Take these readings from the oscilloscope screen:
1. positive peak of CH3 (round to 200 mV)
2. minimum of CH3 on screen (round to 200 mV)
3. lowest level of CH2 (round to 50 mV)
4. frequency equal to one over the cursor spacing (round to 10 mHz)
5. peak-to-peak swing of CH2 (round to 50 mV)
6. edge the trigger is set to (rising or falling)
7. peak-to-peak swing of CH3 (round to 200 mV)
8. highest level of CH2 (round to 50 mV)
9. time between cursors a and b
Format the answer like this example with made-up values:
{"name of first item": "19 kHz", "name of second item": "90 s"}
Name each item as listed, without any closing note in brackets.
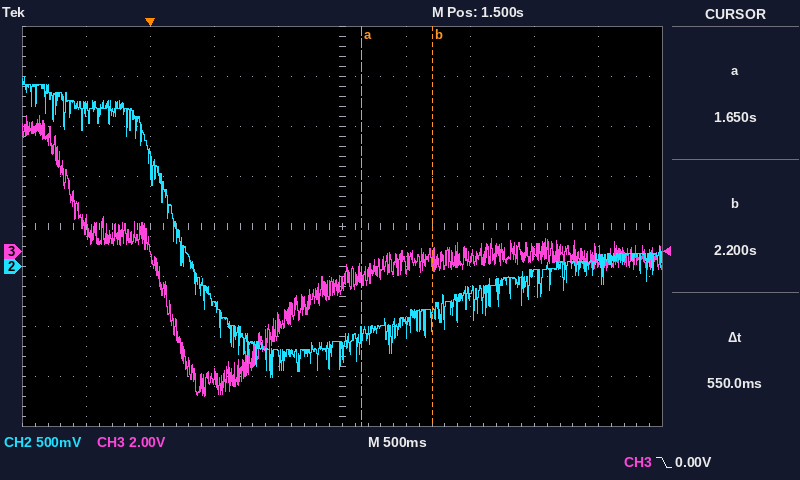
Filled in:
{"positive peak of CH3": "5.4 V", "minimum of CH3 on screen": "-5.8 V", "lowest level of CH2": "-1.10 V", "frequency equal to one over the cursor spacing": "1.82 Hz", "peak-to-peak swing of CH2": "3.00 V", "edge the trigger is set to": "falling", "peak-to-peak swing of CH3": "11.2 V", "highest level of CH2": "1.90 V", "time between cursors a and b": "550 ms"}
